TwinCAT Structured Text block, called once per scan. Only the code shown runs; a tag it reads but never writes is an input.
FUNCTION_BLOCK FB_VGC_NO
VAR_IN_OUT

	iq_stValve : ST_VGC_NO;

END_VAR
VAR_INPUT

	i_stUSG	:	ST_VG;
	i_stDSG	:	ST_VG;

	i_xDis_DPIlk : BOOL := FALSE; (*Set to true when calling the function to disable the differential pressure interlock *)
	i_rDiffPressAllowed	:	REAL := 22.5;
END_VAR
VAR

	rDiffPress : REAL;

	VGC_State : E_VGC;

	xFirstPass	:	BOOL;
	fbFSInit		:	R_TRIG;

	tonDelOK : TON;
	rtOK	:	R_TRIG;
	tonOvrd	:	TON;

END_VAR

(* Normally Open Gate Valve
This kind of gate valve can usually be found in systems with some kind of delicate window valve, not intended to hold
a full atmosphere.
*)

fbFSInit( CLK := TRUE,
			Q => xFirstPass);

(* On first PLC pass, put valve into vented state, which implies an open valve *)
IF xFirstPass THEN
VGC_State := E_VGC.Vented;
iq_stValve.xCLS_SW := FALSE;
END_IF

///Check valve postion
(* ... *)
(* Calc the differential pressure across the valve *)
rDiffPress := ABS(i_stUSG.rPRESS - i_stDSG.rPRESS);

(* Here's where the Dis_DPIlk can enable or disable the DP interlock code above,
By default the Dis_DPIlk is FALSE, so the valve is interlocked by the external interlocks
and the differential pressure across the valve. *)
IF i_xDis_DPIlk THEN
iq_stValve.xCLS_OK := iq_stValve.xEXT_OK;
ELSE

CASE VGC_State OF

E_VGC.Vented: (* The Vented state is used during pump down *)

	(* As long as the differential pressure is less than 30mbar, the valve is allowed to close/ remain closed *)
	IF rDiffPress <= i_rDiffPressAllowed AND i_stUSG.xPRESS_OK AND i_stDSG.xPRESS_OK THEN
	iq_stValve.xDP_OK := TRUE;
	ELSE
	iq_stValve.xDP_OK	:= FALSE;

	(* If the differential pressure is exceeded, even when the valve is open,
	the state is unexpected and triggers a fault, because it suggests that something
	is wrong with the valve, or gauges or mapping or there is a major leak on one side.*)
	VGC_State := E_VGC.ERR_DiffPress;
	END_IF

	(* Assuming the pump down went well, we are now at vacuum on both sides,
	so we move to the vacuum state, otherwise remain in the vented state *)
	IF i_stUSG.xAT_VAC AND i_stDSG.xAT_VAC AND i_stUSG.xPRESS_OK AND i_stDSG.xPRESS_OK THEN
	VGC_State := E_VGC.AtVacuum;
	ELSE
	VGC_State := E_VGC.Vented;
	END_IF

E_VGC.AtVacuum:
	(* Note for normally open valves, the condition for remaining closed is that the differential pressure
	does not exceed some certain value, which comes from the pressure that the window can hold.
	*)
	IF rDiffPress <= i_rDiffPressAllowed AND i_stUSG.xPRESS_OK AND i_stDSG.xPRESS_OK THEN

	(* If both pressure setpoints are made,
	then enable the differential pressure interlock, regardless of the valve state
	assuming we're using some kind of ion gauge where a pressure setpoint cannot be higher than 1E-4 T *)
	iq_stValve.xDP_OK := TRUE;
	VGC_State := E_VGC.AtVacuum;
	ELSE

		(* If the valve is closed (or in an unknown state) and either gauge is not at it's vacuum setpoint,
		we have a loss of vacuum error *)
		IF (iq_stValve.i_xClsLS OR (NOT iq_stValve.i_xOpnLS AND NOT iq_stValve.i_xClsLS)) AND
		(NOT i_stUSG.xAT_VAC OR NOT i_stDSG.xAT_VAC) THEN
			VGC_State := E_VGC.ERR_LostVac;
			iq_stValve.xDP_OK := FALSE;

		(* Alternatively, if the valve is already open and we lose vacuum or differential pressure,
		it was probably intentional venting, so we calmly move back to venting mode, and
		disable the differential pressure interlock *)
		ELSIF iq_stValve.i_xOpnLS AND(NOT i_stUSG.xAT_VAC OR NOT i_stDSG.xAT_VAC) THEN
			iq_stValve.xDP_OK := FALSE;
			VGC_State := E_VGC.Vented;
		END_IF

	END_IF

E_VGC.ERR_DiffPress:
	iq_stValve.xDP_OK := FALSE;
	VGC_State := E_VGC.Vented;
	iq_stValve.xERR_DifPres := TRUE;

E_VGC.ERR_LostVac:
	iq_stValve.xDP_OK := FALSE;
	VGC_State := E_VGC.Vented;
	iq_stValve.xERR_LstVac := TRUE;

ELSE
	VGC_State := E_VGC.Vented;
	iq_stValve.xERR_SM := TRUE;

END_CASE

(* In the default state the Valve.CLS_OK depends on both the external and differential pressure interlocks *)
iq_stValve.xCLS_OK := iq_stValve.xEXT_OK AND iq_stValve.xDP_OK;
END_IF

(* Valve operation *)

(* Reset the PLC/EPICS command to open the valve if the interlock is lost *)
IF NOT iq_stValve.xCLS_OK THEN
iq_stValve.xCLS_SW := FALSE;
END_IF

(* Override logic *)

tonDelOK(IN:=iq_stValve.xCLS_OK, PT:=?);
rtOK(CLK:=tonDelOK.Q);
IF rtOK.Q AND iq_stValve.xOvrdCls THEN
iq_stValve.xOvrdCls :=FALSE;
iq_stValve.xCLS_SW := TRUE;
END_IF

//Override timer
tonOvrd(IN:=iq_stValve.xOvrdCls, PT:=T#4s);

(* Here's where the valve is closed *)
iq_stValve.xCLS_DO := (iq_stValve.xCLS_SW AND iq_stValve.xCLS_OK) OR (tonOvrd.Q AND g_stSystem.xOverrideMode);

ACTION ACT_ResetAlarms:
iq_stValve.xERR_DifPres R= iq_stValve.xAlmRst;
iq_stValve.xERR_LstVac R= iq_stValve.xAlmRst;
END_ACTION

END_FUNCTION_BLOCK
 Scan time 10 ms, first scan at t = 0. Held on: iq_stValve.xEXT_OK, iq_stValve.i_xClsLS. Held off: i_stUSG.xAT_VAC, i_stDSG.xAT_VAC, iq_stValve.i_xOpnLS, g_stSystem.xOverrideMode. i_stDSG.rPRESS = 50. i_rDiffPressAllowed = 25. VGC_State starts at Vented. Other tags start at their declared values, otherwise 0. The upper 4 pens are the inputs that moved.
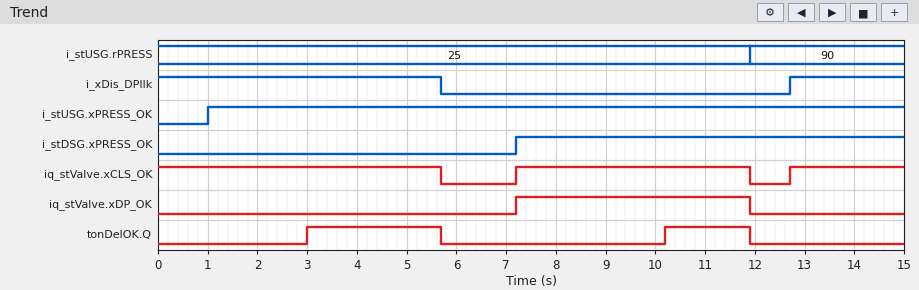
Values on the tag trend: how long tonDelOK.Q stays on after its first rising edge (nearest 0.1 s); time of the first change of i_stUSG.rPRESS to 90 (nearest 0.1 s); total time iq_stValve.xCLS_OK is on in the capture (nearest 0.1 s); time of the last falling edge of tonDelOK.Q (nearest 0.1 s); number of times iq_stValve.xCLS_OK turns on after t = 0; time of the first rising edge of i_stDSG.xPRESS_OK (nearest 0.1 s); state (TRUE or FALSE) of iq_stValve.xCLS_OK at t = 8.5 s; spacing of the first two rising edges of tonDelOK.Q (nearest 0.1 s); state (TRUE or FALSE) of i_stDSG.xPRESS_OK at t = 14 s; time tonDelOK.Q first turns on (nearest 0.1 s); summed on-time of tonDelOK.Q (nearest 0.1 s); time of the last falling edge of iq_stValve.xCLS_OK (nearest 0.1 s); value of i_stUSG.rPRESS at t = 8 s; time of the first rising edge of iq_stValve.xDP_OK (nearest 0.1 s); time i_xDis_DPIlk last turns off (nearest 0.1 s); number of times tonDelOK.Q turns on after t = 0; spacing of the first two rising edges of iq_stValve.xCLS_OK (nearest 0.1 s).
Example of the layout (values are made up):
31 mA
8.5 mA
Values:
2.7 s
11.9 s
12.7 s
11.9 s
2
7.2 s
TRUE
7.2 s
TRUE
3.0 s
4.4 s
11.9 s
25
7.2 s
5.7 s
2
5.5 s
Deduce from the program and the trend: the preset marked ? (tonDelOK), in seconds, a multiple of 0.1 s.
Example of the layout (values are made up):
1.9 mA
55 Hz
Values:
3.0 s
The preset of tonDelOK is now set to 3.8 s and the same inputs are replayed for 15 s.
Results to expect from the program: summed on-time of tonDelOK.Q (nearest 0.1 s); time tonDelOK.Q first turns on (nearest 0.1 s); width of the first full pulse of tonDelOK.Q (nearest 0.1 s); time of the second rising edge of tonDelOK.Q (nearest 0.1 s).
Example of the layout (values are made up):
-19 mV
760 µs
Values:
2.8 s
3.8 s
1.9 s
11.0 s
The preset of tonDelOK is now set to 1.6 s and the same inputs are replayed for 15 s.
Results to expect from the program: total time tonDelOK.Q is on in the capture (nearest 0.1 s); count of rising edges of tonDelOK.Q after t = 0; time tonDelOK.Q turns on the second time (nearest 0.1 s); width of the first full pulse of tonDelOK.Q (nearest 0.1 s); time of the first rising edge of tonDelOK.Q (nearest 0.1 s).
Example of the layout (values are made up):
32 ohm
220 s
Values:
7.9 s
3
8.8 s
4.1 s
1.6 s
